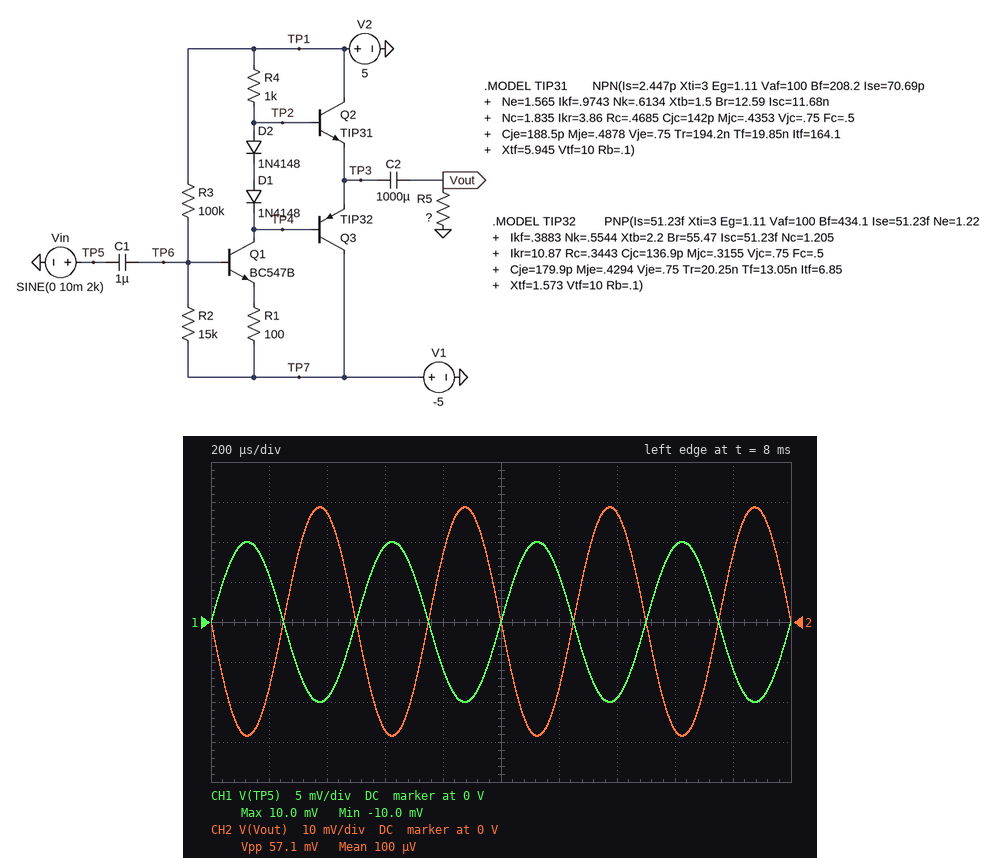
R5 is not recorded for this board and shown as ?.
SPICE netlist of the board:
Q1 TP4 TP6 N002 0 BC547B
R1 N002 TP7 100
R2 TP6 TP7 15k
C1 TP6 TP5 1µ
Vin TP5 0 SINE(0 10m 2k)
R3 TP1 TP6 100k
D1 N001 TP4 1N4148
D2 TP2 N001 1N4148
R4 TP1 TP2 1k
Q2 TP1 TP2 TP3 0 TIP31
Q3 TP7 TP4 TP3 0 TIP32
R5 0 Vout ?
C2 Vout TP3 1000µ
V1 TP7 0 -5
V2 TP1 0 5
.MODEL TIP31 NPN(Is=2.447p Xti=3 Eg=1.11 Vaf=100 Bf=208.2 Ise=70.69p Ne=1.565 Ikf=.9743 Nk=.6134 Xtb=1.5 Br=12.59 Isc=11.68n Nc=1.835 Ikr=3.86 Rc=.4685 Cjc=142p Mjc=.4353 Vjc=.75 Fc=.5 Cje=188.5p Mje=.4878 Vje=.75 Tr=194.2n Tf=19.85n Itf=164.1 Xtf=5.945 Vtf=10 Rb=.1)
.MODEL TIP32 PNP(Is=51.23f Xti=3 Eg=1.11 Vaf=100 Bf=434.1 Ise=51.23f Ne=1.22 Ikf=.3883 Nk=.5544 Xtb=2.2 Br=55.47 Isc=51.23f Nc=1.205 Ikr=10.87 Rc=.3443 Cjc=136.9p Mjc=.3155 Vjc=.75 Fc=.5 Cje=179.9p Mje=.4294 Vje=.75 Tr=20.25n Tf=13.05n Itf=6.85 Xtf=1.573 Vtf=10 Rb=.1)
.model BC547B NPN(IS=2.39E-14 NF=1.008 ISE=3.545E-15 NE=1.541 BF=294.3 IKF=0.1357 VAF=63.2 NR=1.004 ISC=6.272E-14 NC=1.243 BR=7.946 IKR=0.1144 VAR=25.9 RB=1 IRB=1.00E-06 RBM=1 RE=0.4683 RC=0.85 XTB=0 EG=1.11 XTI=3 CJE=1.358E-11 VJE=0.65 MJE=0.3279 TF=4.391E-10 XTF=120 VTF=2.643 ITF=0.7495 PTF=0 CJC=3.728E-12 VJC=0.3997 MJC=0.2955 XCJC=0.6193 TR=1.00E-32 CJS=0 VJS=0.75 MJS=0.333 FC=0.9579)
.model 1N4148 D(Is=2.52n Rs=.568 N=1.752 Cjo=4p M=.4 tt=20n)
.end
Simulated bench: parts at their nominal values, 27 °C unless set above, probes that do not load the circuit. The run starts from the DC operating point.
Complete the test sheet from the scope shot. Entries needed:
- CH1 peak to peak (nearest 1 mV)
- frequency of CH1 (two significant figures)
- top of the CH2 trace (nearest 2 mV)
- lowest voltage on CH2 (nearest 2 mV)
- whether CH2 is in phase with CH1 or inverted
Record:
20 mV
2.0 kHz
28 mV
-28 mV
inverted
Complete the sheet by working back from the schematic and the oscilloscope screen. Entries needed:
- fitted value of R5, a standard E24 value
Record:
4.3 Ω
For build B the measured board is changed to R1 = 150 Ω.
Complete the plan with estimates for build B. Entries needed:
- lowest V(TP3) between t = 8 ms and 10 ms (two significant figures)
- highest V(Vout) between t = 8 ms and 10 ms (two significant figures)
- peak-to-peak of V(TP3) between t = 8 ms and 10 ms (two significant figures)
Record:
1.1 V
19 mV
37 mV
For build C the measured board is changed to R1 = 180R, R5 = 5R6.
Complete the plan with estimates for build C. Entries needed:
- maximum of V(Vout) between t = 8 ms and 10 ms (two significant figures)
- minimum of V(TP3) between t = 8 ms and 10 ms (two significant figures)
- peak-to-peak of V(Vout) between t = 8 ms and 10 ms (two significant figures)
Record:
18 mV
1.5 V
36 mV
